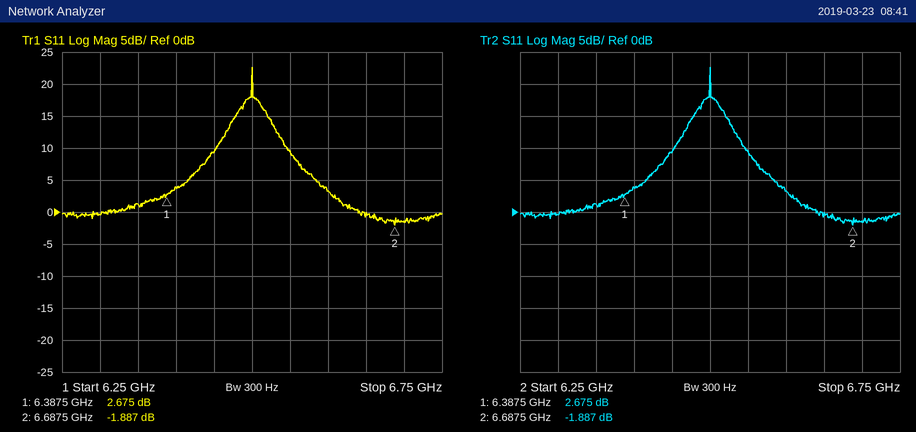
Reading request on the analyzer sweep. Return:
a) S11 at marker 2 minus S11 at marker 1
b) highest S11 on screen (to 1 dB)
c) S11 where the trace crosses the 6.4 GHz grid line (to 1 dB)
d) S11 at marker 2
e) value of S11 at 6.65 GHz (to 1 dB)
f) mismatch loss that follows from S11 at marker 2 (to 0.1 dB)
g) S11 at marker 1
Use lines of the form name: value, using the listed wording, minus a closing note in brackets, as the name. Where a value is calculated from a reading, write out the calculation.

S11 at marker 2 minus S11 at marker 1: -1.887 − (2.675) = -4.562 dB
highest S11 on screen: 23 dB
S11 where the trace crosses the 6.4 GHz grid line: 4 dB
S11 at marker 2: -1.887 dB
value of S11 at 6.65 GHz: 0 dB
mismatch loss that follows from S11 at marker 2: −10 log10(1 − 10^(-1.887/10)) ≈ 4.5 dB
S11 at marker 1: 2.675 dB
